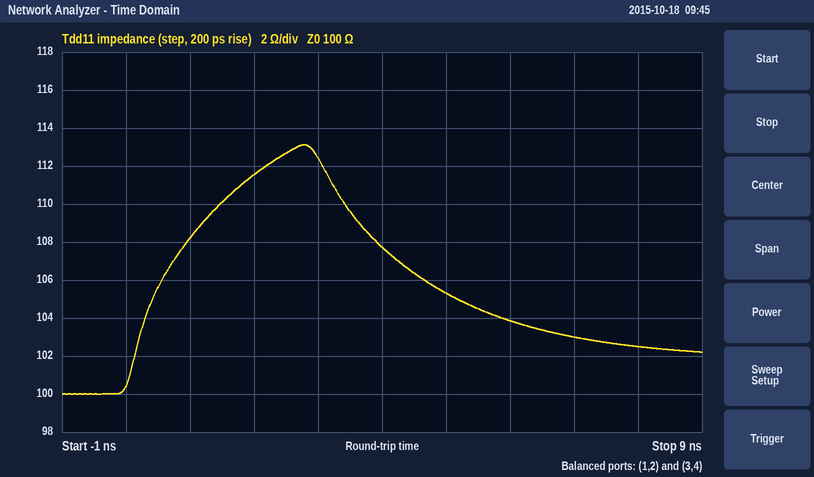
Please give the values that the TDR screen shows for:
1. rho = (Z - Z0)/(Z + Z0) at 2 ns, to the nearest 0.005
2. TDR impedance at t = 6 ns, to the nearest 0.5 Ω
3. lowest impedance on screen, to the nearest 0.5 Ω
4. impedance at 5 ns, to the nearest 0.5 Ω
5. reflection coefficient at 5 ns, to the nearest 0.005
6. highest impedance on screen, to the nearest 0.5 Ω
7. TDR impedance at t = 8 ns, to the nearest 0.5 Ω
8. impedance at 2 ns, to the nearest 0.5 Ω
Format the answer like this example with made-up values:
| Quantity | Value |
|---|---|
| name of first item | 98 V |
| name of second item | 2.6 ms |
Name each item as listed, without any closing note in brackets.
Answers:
| Quantity | Value |
|---|---|
| rho = (Z - Z0)/(Z + Z0) at 2 ns, to the nearest 0.005 | +0.055 |
| TDR impedance at t = 6 ns, to the nearest 0.5 Ω | 104.0 Ω |
| lowest impedance on screen, to the nearest 0.5 Ω | 100.0 Ω |
| impedance at 5 ns, to the nearest 0.5 Ω | 105.5 Ω |
| reflection coefficient at 5 ns, to the nearest 0.005 | +0.025 |
| highest impedance on screen, to the nearest 0.5 Ω | 113.0 Ω |
| TDR impedance at t = 8 ns, to the nearest 0.5 Ω | 102.5 Ω |
| impedance at 2 ns, to the nearest 0.5 Ω | 111.5 Ω |
